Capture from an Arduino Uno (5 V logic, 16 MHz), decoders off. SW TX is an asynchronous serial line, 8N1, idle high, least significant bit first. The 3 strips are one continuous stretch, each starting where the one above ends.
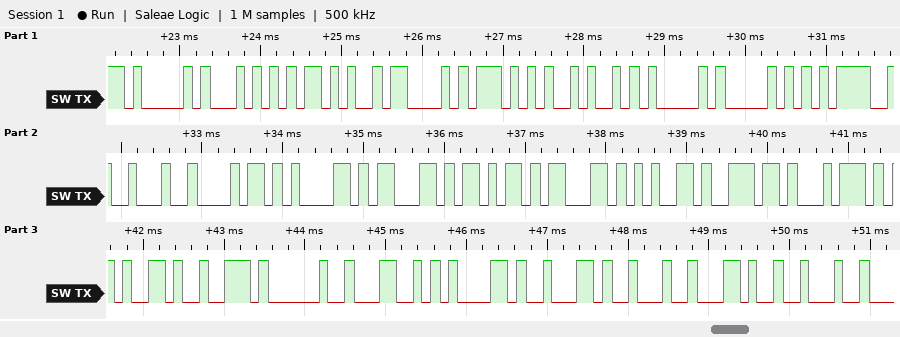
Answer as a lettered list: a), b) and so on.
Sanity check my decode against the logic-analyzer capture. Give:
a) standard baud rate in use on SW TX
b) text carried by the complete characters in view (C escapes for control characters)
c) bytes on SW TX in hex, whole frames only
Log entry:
a) 9600 baud
b) "AT+CWJAP=\"hackcenter Lab\",\""
c) 0x41 0x54 0x2B 0x43 0x57 0x4A 0x41 0x50 0x3D 0x22 0x68 0x61 0x63 0x6B 0x63 0x65 0x6E 0x74 0x65 0x72 0x20 0x4C 0x61 0x62 0x22 0x2C 0x22
